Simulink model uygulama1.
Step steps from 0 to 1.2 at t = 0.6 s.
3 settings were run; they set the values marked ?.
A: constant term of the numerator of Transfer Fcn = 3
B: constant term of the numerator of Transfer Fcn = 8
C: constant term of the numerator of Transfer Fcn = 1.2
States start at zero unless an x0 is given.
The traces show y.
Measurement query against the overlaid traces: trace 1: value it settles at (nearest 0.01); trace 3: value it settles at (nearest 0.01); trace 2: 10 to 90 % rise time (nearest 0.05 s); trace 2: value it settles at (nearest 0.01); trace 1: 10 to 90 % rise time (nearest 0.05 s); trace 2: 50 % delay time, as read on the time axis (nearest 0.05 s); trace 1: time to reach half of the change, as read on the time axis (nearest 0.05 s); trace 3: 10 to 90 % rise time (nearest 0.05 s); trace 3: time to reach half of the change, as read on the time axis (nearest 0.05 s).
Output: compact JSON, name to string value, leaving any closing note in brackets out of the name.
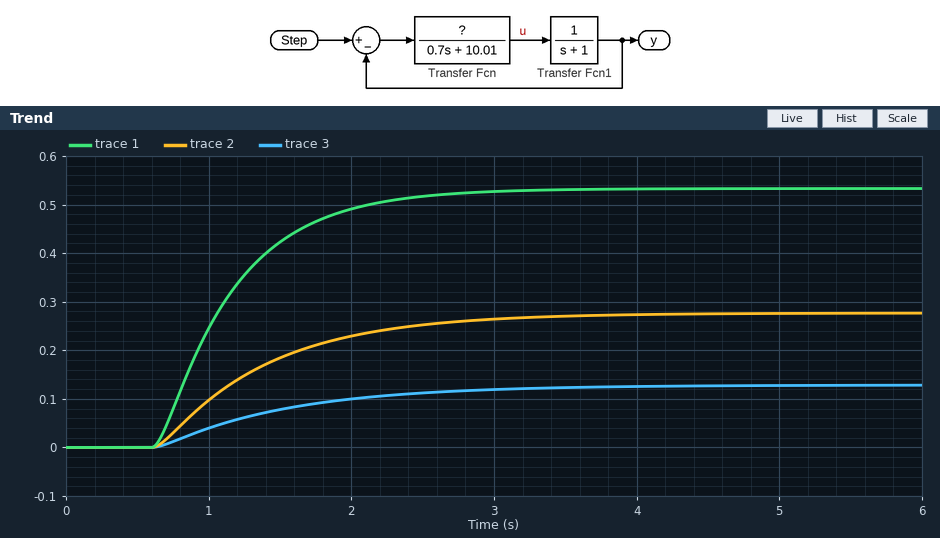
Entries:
{"trace 1: value it settles at": "0.53", "trace 3: value it settles at": "0.13", "trace 2: 10 to 90 % rise time": "1.65 s", "trace 2: value it settles at": "0.28", "trace 1: 10 to 90 % rise time": "1.15 s", "trace 2: 50 % delay time, as read on the time axis": "1.20 s", "trace 1: time to reach half of the change, as read on the time axis": "1.05 s", "trace 3: 10 to 90 % rise time": "1.95 s", "trace 3: time to reach half of the change, as read on the time axis": "1.30 s"}
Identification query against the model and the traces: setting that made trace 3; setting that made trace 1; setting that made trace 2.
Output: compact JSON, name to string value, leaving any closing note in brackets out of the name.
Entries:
{"setting that made trace 3": "C", "setting that made trace 1": "B", "setting that made trace 2": "A"}
